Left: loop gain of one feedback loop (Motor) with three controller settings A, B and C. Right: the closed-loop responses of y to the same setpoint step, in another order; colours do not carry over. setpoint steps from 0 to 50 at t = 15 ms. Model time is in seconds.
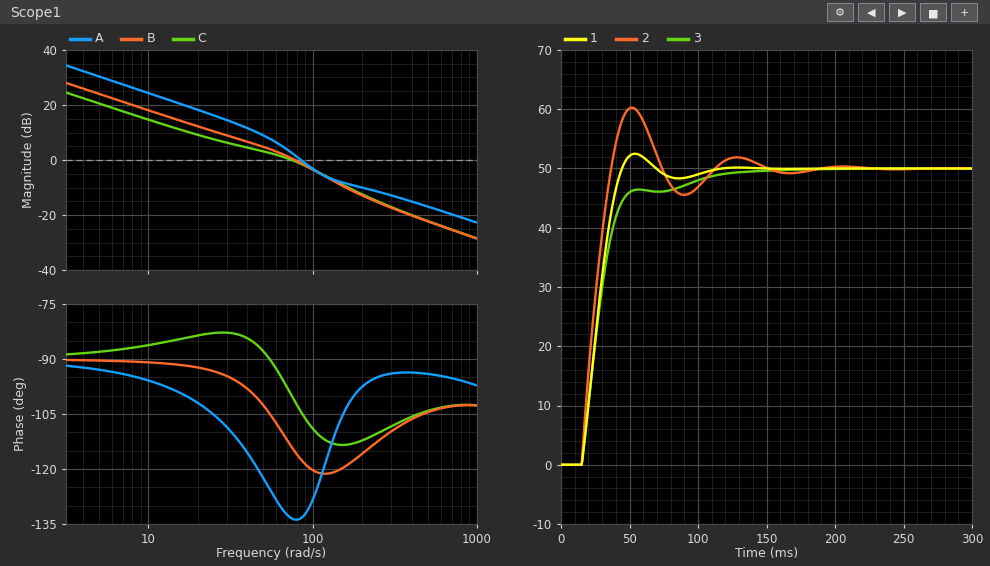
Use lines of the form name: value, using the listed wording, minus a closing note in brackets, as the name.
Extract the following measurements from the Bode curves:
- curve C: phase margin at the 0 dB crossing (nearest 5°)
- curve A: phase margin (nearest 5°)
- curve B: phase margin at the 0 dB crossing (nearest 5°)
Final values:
curve C: phase margin at the 0 dB crossing: 80°
curve A: phase margin: 45°
curve B: phase margin at the 0 dB crossing: 65°
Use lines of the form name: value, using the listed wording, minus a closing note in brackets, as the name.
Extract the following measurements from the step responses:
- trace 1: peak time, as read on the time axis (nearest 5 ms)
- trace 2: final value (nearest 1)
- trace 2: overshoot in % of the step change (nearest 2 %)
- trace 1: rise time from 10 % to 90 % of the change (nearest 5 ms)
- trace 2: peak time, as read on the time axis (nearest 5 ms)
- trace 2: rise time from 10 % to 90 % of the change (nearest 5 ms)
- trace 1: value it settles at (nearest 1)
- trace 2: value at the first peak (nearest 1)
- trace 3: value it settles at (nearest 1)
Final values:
trace 1: peak time, as read on the time axis: 55 ms
trace 2: final value: 50
trace 2: overshoot in % of the step change: 20 %
trace 1: rise time from 10 % to 90 % of the change: 20 ms
trace 2: peak time, as read on the time axis: 50 ms
trace 2: rise time from 10 % to 90 % of the change: 15 ms
trace 1: value it settles at: 50
trace 2: value at the first peak: 60
trace 3: value it settles at: 50
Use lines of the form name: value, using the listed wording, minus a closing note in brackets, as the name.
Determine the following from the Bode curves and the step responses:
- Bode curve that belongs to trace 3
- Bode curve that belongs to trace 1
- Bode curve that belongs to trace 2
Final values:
Bode curve that belongs to trace 3: C
Bode curve that belongs to trace 1: B
Bode curve that belongs to trace 2: A
